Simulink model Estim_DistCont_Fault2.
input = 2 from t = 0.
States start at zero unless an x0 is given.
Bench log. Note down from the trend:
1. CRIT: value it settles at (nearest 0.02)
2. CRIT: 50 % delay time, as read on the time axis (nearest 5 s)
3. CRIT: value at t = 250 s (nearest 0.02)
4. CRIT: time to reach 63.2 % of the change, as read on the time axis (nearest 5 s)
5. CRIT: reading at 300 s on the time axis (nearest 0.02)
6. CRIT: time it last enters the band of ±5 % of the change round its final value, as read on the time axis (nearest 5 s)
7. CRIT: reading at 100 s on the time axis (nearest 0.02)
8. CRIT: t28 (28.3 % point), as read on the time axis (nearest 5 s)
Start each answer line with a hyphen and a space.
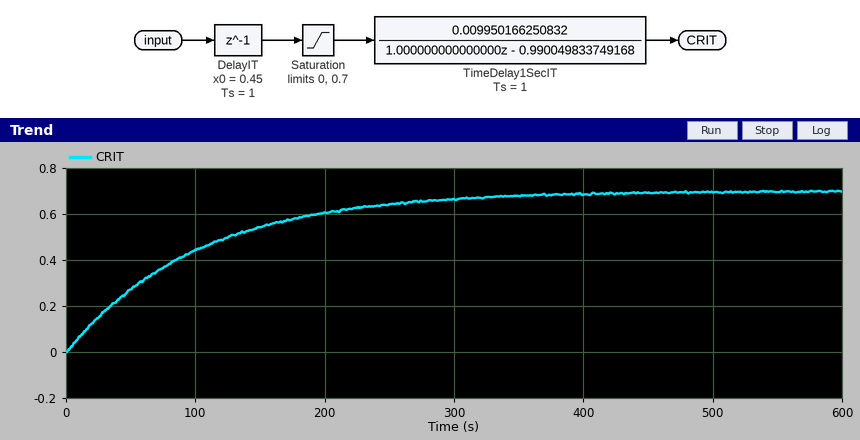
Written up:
- 0.70
- 70 s
- 0.64
- 100 s
- 0.66
- 300 s
- 0.44
- 35 s
